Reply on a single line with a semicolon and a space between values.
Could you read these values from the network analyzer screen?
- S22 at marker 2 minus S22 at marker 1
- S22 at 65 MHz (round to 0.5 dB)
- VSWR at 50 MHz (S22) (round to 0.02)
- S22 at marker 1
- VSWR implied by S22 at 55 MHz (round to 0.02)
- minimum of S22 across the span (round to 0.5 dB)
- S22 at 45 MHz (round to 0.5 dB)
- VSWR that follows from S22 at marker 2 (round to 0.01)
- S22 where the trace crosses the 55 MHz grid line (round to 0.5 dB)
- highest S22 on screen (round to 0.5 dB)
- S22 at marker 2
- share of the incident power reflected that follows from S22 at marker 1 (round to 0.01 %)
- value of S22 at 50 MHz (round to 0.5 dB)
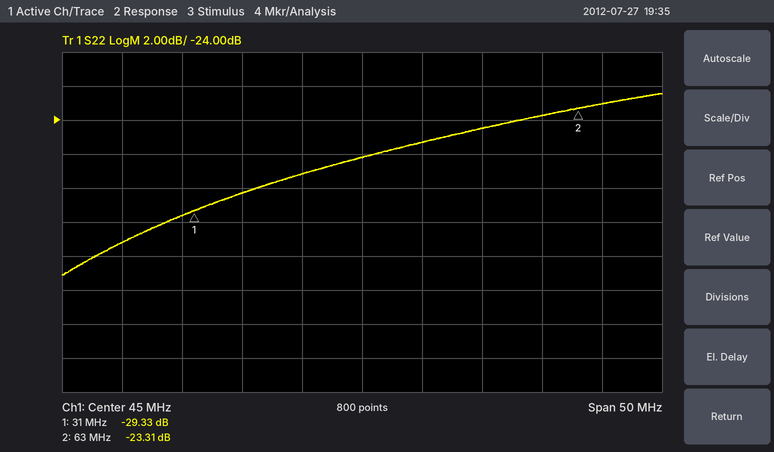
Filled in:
6.02 dB; -23.0 dB; 1.12; -29.33 dB; 1.12; -33.0 dB; -26.0 dB; 1.15; -24.5 dB; -22.5 dB; -23.31 dB; 0.12 %; -25.5 dB
